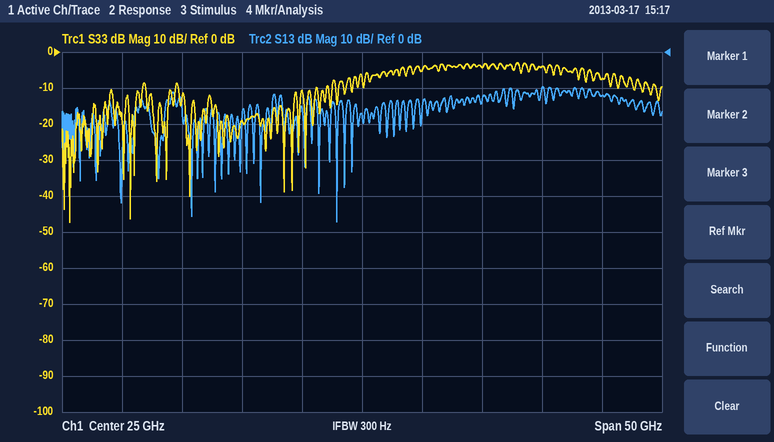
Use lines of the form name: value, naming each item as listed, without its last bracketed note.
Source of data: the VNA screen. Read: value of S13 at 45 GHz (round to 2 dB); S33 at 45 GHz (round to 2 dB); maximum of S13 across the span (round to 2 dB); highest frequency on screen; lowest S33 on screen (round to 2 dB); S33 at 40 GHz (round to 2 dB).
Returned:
value of S13 at 45 GHz: -12 dB
S33 at 45 GHz: -8 dB
maximum of S13 across the span: -10 dB
highest frequency on screen: 50 GHz
lowest S33 on screen: -48 dB
S33 at 40 GHz: -4 dB
